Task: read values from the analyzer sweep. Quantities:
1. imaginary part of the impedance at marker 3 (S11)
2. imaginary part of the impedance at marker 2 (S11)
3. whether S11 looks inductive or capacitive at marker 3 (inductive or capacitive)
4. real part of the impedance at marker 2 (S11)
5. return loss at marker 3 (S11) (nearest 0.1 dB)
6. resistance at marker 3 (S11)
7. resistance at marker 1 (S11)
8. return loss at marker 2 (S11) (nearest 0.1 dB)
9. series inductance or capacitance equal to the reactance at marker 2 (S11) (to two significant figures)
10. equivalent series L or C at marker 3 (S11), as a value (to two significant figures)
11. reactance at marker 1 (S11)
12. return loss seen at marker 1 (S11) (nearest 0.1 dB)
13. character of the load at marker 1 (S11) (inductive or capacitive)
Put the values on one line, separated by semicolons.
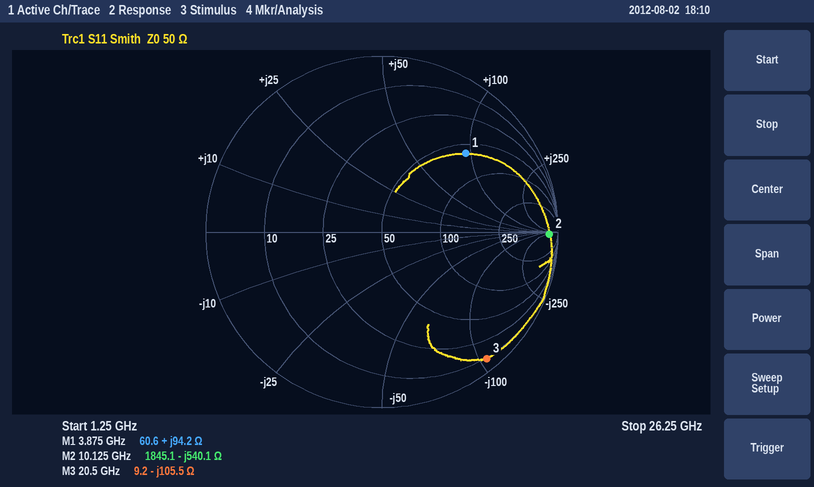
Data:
-105.5 Ω; -540.1 Ω; capacitive; 1845.1 Ω; 0.6 dB; 9.2 Ω; 60.6 Ω; 0.4 dB; 29 fF; 74 fF; +94.2 Ω; 3.7 dB; inductive
